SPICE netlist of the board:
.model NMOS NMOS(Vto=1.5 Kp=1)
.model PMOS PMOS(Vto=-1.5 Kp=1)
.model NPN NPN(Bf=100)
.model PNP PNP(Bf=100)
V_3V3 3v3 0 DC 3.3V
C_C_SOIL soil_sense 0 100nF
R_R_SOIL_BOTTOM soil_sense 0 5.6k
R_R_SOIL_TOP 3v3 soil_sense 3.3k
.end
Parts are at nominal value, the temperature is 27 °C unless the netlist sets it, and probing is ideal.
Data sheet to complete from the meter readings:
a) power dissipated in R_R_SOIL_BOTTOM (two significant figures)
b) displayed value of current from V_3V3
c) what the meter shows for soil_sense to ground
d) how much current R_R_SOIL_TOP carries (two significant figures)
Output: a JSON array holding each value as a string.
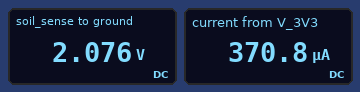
["770 µW", "370.8 µA", "2.076 V", "370 µA"]
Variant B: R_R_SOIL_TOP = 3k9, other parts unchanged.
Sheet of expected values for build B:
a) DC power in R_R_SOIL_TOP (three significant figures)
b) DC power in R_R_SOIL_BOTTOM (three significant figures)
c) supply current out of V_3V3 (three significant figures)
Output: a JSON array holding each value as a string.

["471 µW", "676 µW", "347 µA"]
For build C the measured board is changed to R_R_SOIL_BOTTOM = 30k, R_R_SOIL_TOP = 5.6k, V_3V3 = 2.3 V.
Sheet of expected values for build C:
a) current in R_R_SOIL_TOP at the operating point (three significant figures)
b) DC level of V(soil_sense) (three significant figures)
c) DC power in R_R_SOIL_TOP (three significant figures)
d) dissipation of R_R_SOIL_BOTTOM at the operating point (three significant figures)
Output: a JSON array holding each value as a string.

["64.6 µA", "1.94 V", "23.4 µW", "125 µW"]
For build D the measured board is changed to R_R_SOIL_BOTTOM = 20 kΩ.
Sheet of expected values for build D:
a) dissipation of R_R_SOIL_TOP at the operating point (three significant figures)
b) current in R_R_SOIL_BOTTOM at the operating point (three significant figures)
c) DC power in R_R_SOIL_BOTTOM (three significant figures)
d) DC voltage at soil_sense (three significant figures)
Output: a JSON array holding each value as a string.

["66.2 µW", "142 µA", "401 µW", "2.83 V"]
